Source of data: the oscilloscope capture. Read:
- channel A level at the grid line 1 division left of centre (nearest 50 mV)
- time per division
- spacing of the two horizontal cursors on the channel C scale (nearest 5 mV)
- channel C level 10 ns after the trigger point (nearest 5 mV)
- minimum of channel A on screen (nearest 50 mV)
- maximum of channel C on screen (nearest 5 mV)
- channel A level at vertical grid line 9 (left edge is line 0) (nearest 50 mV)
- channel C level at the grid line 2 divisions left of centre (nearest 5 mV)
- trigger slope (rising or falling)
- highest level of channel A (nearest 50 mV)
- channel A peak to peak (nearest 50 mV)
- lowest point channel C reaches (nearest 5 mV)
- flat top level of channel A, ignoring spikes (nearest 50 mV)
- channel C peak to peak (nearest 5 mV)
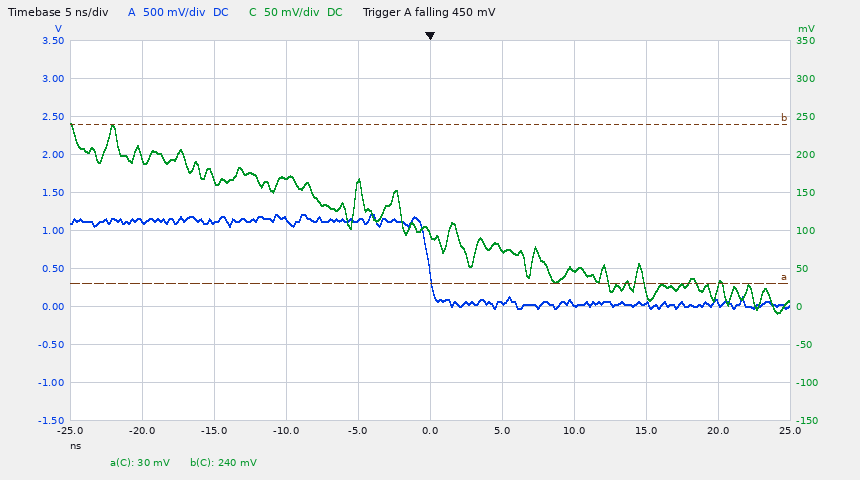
1.15 V
5 ns
210 mV
50 mV
-50 mV
240 mV
50 mV
170 mV
falling
1.20 V
1.25 V
-10 mV
1.15 V
250 mV
